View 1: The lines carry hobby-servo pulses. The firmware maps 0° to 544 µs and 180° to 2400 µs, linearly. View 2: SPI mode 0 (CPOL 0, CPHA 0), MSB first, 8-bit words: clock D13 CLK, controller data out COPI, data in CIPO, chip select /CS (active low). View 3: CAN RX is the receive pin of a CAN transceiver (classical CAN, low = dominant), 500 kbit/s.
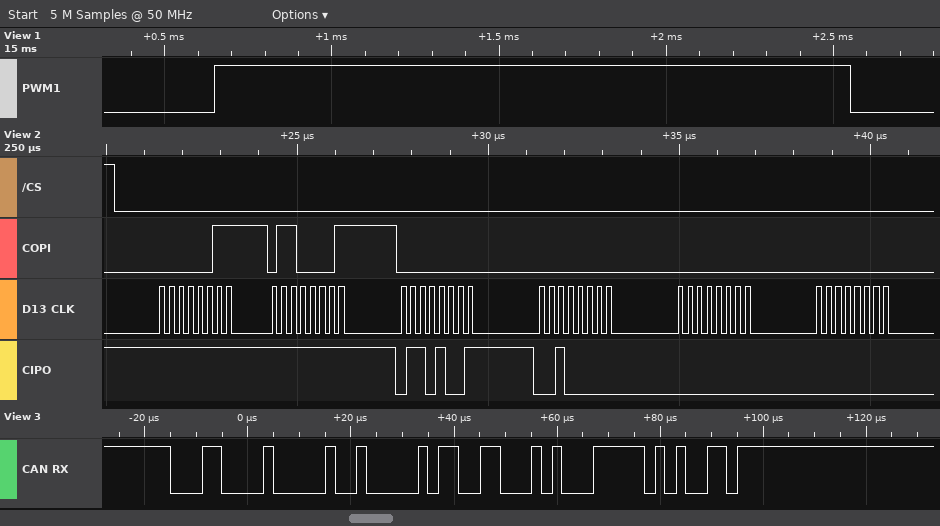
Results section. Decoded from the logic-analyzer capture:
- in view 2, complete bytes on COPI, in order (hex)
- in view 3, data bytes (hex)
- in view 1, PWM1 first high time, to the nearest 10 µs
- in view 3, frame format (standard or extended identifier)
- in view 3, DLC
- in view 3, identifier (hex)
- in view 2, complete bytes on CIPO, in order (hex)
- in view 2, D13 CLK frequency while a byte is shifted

03 61 00 00 00 00
06 62
1900 µs
standard
2
0x184
FF FF 69 20 00 00
4 MHz
